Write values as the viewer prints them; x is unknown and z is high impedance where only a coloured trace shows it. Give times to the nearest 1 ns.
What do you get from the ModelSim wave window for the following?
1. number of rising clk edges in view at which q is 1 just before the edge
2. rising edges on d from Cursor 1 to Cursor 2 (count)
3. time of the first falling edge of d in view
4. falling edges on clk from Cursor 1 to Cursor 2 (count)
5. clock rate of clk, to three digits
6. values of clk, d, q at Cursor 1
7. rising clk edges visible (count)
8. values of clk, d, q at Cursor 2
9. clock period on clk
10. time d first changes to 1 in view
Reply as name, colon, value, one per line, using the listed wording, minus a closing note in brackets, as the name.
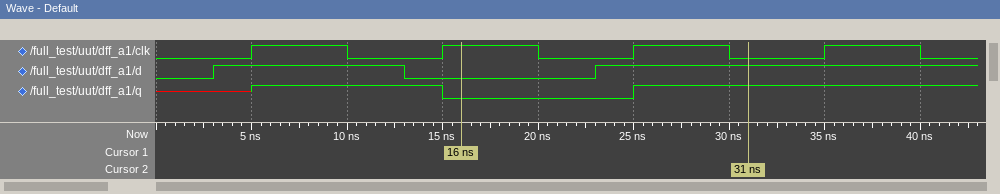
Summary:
number of rising clk edges in view at which q is 1 just before the edge: 2
rising edges on d from Cursor 1 to Cursor 2: 1
time of the first falling edge of d in view: 13 ns
falling edges on clk from Cursor 1 to Cursor 2: 2
clock rate of clk, to three digits: 100 MHz
values of clk, d, q at Cursor 1: clk=1, d=0, q=0
rising clk edges visible: 4
values of clk, d, q at Cursor 2: clk=0, d=1, q=1
clock period on clk: 10 ns
time d first changes to 1 in view: 3 ns
